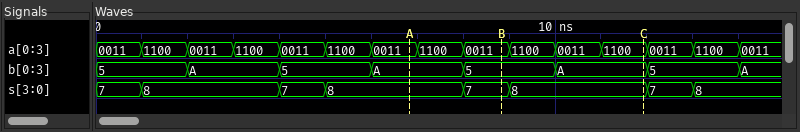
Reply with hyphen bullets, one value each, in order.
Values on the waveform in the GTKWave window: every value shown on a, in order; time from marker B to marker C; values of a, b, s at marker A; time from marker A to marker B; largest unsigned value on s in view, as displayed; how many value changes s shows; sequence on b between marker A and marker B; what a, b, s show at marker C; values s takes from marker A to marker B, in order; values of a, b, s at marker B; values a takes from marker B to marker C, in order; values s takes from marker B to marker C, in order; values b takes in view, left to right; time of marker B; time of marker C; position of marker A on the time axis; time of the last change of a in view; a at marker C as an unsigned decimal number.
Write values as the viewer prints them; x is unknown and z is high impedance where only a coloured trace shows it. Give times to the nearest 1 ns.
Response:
- 0011, 1100, 0011, 1100, 0011, 1100, 0011, 1100, 0011, 1100, 0011, 1100, 0011, 1100, 0011
- 3 ns
- a=0011, b=A, s=8
- 2 ns
- 8
- 7
- A, 5
- a=1100, b=A, s=8
- 8, 7
- a=0011, b=5, s=7
- 0011, 1100, 0011, 1100
- 7, 8
- 5, A, 5, A, 5, A, 5, A
- 9 ns
- 12 ns
- 7 ns
- 14 ns
- 12
